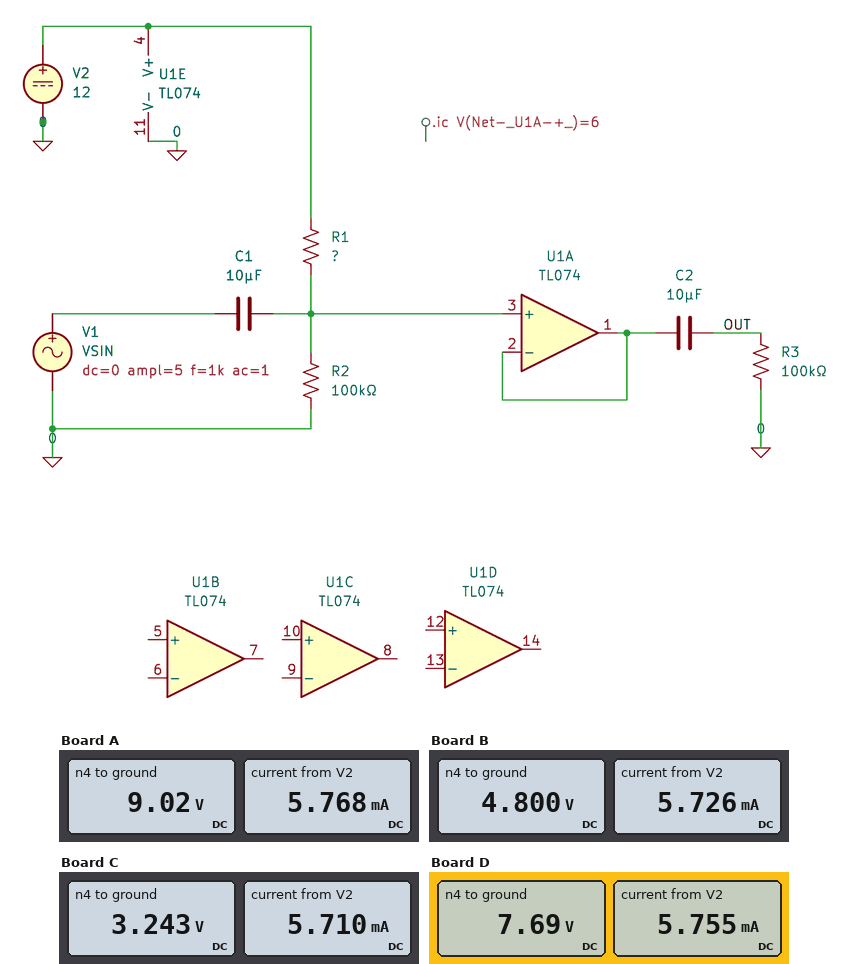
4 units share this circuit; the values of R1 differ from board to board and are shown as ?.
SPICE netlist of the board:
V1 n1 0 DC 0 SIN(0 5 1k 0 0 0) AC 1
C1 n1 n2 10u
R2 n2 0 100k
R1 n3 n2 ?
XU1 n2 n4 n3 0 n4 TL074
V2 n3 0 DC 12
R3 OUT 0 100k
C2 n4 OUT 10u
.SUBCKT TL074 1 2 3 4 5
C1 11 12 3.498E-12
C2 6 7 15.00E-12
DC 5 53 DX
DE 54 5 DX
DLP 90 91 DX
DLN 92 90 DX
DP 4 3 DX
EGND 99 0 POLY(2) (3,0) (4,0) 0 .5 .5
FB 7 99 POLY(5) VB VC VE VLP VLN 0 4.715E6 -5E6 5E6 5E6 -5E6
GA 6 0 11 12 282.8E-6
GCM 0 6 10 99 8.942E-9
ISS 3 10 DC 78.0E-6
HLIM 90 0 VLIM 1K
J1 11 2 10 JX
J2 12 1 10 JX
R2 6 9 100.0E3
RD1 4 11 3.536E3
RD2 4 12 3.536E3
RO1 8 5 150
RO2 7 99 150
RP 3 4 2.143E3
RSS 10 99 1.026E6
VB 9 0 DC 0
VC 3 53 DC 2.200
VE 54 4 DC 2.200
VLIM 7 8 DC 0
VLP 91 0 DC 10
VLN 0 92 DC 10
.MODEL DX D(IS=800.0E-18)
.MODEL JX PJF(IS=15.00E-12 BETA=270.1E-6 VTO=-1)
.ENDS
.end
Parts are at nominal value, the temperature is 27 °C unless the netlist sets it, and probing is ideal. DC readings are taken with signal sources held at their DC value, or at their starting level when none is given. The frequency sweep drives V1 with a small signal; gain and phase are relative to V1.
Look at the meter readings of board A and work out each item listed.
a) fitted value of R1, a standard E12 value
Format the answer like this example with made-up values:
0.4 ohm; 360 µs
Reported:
33 kΩ
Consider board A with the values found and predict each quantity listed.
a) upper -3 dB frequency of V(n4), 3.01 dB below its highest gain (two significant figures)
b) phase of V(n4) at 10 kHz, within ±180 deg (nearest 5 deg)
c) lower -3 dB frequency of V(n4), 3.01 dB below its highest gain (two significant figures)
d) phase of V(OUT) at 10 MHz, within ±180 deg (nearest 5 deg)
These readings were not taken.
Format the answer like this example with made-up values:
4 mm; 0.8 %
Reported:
2.9 MHz; 0 deg; 640 mHz; -145 deg
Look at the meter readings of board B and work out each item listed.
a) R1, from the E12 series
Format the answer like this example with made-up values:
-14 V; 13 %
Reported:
150 kΩ
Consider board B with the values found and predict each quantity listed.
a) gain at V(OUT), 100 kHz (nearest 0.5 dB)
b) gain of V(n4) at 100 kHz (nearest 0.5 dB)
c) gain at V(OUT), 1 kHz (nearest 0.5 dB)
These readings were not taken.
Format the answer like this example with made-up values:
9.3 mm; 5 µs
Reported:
0 dB; 0 dB; 0 dB
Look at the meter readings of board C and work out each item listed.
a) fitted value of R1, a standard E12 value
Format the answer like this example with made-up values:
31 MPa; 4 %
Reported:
270 kΩ
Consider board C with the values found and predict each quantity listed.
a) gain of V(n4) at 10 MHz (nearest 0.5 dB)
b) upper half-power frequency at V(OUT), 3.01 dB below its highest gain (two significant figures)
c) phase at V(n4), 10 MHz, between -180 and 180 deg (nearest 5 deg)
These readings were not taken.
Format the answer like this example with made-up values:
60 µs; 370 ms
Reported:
-17.5 dB; 3.0 MHz; -145 deg
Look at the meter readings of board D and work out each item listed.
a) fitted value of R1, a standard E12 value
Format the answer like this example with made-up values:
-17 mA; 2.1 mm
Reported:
56 kΩ
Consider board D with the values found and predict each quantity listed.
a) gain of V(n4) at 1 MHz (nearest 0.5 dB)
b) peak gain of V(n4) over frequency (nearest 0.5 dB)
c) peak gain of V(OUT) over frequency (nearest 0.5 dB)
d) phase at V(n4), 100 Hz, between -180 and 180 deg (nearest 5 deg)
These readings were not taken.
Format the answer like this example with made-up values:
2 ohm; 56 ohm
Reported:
-0.5 dB; 0 dB; 0 dB; 0 deg
